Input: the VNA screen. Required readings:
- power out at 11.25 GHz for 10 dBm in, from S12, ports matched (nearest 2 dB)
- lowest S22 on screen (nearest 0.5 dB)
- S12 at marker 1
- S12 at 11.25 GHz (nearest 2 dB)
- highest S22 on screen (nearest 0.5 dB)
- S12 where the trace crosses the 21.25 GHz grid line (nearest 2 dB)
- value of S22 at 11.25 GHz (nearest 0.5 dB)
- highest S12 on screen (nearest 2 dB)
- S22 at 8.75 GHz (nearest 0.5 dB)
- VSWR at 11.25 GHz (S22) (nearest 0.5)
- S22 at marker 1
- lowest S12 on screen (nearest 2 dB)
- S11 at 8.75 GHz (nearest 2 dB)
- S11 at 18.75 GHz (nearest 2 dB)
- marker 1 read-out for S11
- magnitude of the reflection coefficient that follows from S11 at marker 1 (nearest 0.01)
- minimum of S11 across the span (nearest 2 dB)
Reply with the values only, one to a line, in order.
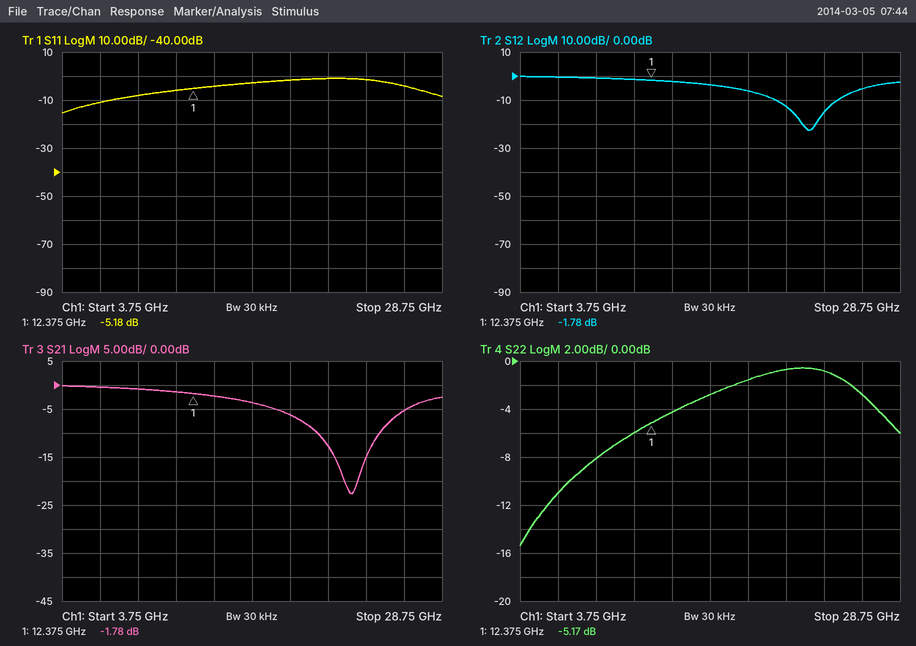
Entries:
8 dBm
-15.5 dB
-1.78 dB
-2 dB
-0.5 dB
-12 dB
-6.0 dB
0 dB
-8.0 dB
3.0
-5.17 dB
-22 dB
-8 dB
-2 dB
-5.18 dB
0.55
-16 dB
